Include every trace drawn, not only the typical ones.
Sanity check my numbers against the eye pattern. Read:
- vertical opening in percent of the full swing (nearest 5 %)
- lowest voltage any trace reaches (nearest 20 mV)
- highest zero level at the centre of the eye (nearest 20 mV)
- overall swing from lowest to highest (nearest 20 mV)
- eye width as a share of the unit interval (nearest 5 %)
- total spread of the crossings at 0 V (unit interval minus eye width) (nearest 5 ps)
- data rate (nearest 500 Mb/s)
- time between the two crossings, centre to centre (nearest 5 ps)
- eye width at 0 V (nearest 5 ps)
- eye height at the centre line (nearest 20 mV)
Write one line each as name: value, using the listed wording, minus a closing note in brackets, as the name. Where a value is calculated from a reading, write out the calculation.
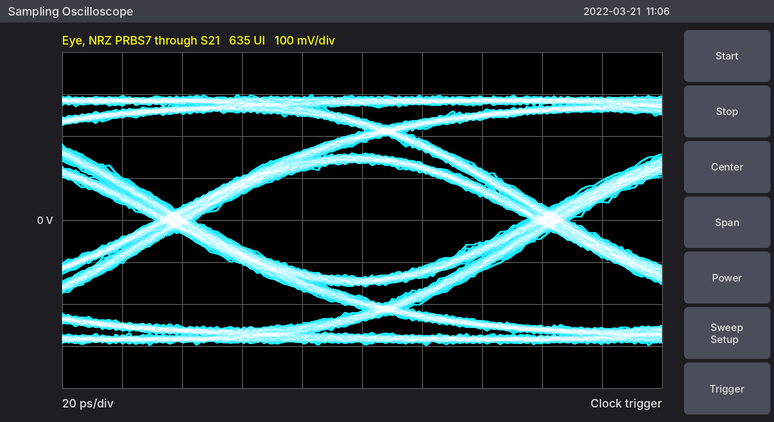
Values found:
vertical opening in percent of the full swing: 280 mV / 600 mV ≈ 46.7 %, so 45 % to the nearest 5 %
lowest voltage any trace reaches: -300 mV
highest zero level at the centre of the eye: -140 mV
overall swing from lowest to highest: 600 mV
eye width as a share of the unit interval: 110 ps / 125 ps ≈ 88.0 %, so 90 % to the nearest 5 %
total spread of the crossings at 0 V (unit interval minus eye width): 15 ps
data rate: 8.0 Gb/s
time between the two crossings, centre to centre: 125 ps
eye width at 0 V: 110 ps
eye height at the centre line: 280 mV
